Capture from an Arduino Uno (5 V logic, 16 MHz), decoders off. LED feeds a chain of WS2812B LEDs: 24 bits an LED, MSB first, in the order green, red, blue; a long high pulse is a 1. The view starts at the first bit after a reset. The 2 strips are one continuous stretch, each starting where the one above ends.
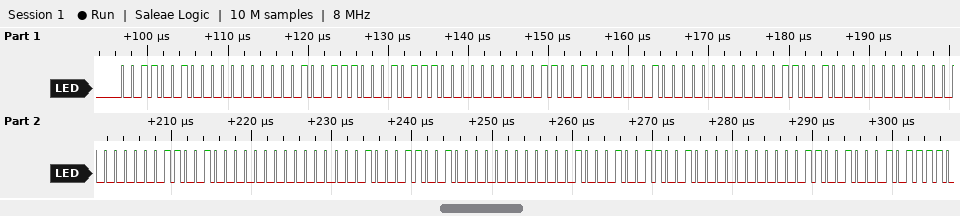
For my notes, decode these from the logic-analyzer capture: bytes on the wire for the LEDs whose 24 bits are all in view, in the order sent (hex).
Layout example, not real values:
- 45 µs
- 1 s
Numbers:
- 32 00 27 17 00 32 04 00 32 00 00 32 00 02 32 00 11 32 00 32 2F
